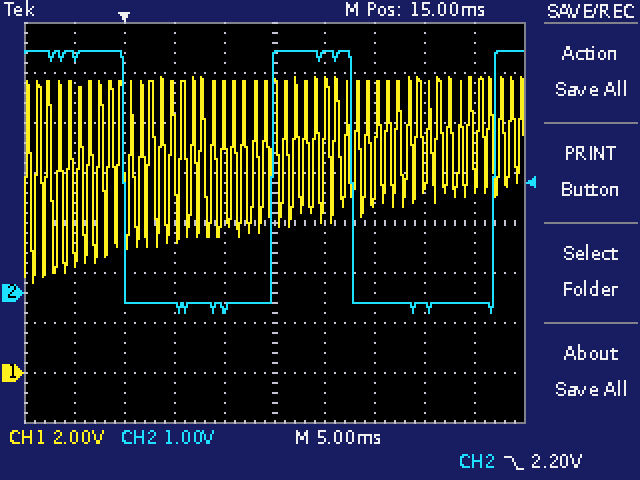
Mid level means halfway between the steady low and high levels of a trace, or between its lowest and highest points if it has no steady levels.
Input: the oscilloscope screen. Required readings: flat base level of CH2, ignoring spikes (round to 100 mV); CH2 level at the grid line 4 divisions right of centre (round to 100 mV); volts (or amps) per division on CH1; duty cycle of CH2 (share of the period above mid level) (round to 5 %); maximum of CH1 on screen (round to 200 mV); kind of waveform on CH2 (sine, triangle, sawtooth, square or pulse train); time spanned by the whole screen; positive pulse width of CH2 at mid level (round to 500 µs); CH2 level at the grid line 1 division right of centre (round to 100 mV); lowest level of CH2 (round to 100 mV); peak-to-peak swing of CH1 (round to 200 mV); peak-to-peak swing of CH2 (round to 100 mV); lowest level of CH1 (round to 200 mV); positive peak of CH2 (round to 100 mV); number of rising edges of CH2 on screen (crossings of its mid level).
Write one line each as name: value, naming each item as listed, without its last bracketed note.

flat base level of CH2, ignoring spikes: -200 mV
CH2 level at the grid line 4 divisions right of centre: -200 mV
volts (or amps) per division on CH1: 2 V
duty cycle of CH2 (share of the period above mid level): 35 %
maximum of CH1 on screen: 11.8 V
kind of waveform on CH2: pulse train
time spanned by the whole screen: 50 ms
positive pulse width of CH2 at mid level: 8.0 ms
CH2 level at the grid line 1 division right of centre: 4.8 V
lowest level of CH2: -400 mV
peak-to-peak swing of CH1: 8.2 V
peak-to-peak swing of CH2: 5.2 V
lowest level of CH1: 3.6 V
positive peak of CH2: 4.8 V
number of rising edges of CH2 on screen: 2
